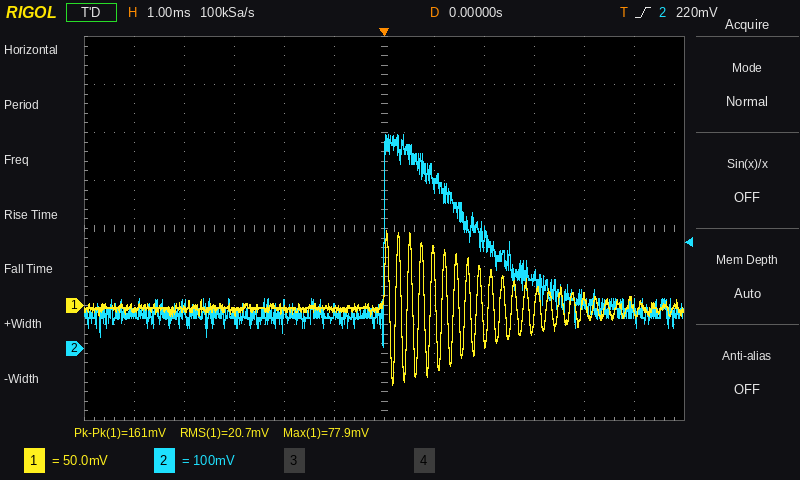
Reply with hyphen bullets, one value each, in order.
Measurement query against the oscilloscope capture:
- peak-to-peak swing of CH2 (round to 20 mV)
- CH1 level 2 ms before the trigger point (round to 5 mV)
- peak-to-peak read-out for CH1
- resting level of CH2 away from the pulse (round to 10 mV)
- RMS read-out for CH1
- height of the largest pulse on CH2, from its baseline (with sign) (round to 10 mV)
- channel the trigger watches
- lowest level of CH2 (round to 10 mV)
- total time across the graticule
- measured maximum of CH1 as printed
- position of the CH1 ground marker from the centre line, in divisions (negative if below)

- 440 mV
- -5 mV
- 161 mV
- 70 mV
- 20.7 mV
- +370 mV
- CH2
- 0 mV
- 12 ms
- 77.9 mV
- -1.6 div
